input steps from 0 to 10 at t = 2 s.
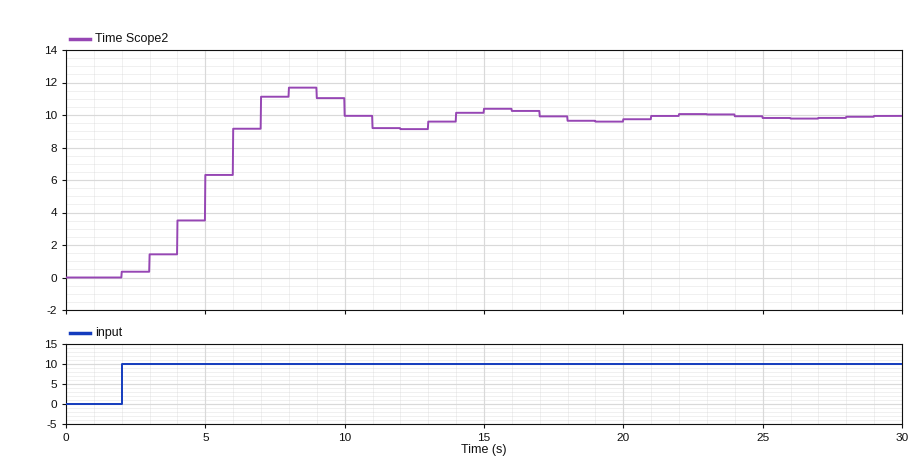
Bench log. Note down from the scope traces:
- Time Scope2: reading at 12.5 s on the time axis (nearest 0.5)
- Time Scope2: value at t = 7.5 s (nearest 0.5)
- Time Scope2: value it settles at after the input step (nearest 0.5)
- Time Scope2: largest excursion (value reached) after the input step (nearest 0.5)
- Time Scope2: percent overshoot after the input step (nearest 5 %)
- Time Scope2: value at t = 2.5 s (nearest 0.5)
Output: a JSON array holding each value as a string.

["9.0", "11.0", "10.0", "11.5", "20 %", "0.5"]
